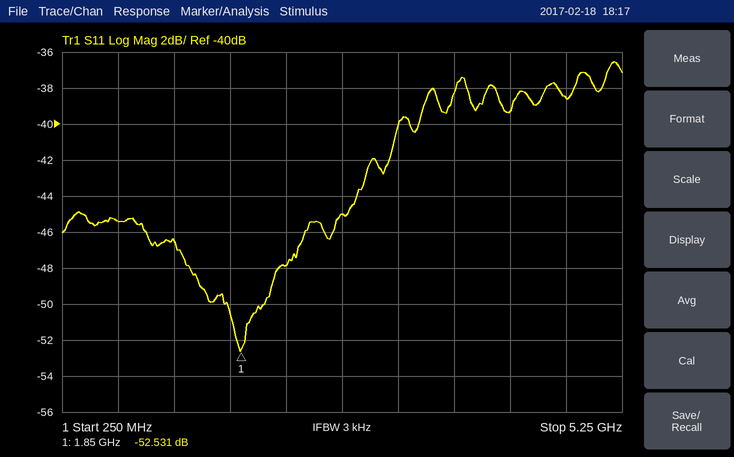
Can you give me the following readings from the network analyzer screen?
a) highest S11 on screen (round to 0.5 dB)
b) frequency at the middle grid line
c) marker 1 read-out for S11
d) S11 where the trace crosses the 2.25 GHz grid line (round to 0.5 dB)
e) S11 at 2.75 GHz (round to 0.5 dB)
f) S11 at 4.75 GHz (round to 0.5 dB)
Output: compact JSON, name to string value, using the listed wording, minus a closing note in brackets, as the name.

{"highest S11 on screen": "-36.5 dB", "frequency at the middle grid line": "2.75 GHz", "marker 1 read-out for S11": "-52.531 dB", "S11 where the trace crosses the 2.25 GHz grid line": "-48.0 dB", "S11 at 2.75 GHz": "-45.0 dB", "S11 at 4.75 GHz": "-38.5 dB"}
